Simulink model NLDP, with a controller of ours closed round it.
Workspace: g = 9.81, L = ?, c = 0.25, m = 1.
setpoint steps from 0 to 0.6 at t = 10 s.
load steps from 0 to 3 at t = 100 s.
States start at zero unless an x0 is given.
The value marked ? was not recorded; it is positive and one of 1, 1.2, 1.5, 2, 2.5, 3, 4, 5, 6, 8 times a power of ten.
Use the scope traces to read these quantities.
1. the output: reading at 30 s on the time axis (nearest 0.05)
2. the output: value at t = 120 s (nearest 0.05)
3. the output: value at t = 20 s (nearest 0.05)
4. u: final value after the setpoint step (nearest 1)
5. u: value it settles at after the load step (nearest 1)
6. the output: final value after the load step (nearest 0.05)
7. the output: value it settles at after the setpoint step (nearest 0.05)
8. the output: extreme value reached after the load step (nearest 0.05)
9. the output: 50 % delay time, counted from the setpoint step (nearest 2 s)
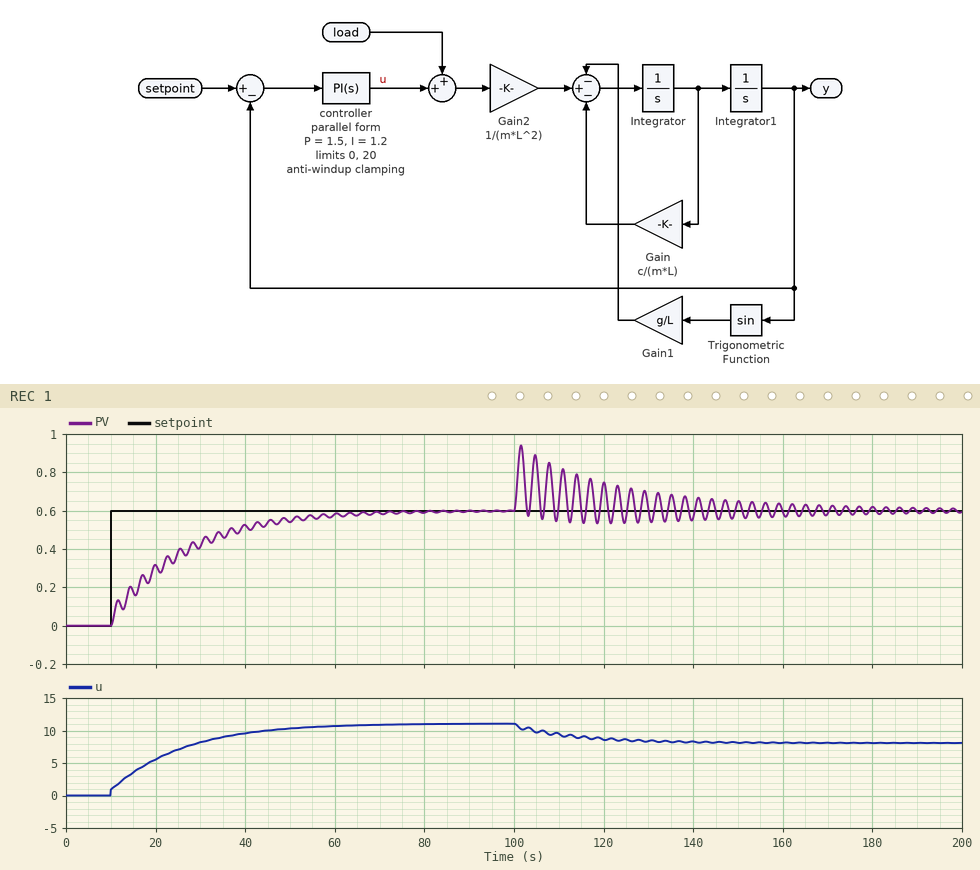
0.40
0.75
0.30
11
8
0.60
0.60
0.95
10 s
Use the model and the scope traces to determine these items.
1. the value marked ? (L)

2
